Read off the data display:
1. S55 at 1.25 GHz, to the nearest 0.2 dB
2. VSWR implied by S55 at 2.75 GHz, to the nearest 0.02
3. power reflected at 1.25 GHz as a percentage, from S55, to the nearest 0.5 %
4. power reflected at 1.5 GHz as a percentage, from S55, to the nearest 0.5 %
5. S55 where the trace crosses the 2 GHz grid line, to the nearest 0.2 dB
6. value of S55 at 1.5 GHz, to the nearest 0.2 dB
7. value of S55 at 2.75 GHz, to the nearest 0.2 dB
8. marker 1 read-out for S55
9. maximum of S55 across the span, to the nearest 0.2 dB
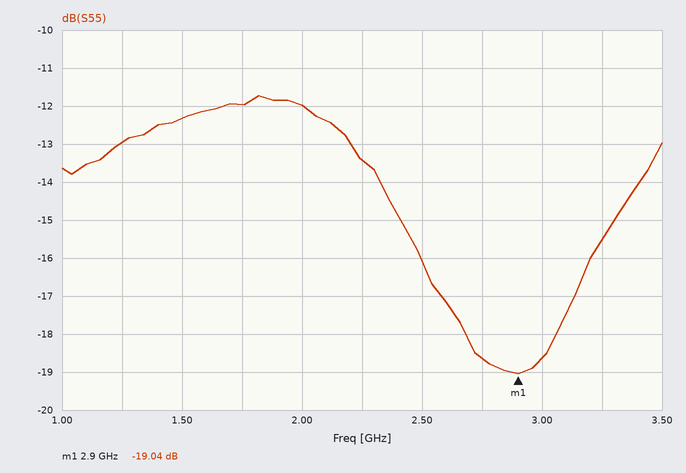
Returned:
-13.0 dB
1.26
5.0 %
6.0 %
-12.0 dB
-12.4 dB
-18.6 dB
-19.04 dB
-11.8 dB
